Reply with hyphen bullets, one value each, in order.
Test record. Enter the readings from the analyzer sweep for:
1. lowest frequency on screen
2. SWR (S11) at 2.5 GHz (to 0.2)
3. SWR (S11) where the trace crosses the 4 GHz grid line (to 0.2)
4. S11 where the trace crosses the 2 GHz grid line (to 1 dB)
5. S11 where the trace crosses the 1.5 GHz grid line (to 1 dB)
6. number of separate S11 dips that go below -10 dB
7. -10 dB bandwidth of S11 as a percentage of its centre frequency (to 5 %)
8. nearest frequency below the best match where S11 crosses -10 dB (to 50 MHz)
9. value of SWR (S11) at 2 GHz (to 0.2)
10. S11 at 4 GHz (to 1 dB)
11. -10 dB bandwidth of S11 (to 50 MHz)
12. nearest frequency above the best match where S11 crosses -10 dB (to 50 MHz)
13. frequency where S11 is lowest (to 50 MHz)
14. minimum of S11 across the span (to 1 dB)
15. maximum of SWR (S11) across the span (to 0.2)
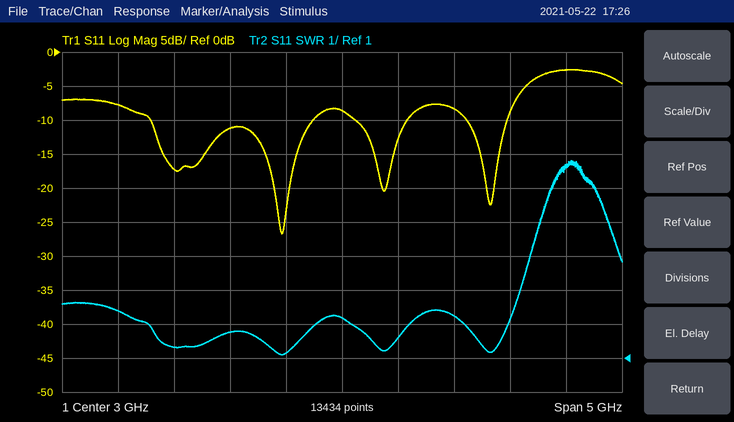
- 500 MHz
- 1.2
- 2.2
- -11 dB
- -17 dB
- 4
- 70 %
- 1.30 GHz
- 1.8
- -8 dB
- 1.45 GHz
- 2.75 GHz
- 2.45 GHz
- -27 dB
- 6.8
